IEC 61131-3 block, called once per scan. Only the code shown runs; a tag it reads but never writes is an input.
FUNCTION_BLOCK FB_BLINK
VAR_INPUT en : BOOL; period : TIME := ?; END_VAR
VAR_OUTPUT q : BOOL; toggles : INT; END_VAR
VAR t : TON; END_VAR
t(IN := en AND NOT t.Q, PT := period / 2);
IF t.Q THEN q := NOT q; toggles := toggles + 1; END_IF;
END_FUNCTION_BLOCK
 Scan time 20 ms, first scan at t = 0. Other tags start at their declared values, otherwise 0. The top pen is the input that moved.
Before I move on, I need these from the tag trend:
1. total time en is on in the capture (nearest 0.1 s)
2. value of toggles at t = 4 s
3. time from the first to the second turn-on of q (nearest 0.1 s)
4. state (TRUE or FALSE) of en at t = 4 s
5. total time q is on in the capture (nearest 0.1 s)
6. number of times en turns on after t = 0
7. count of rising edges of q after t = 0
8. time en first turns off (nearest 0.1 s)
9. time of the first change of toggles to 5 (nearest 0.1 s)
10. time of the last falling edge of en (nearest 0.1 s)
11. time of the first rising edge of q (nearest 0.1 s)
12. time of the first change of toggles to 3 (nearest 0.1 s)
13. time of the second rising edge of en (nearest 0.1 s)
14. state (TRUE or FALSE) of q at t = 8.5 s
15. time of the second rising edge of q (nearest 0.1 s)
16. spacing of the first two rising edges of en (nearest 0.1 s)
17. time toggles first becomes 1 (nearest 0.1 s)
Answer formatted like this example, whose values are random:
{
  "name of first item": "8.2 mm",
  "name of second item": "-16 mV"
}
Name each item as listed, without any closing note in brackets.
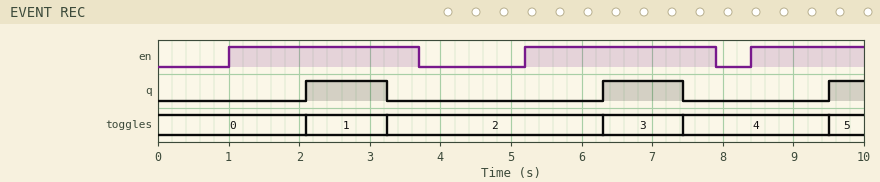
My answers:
{
  "total time en is on in the capture": "7.0 s",
  "value of toggles at t = 4 s": "2",
  "time from the first to the second turn-on of q": "4.2 s",
  "state (TRUE or FALSE) of en at t = 4 s": "FALSE",
  "total time q is on in the capture": "2.8 s",
  "number of times en turns on after t = 0": "3",
  "count of rising edges of q after t = 0": "3",
  "time en first turns off": "3.7 s",
  "time of the first change of toggles to 5": "9.5 s",
  "time of the last falling edge of en": "7.9 s",
  "time of the first rising edge of q": "2.1 s",
  "time of the first change of toggles to 3": "6.3 s",
  "time of the second rising edge of en": "5.2 s",
  "state (TRUE or FALSE) of q at t = 8.5 s": "FALSE",
  "time of the second rising edge of q": "6.3 s",
  "spacing of the first two rising edges of en": "4.2 s",
  "time toggles first becomes 1": "2.1 s"
}
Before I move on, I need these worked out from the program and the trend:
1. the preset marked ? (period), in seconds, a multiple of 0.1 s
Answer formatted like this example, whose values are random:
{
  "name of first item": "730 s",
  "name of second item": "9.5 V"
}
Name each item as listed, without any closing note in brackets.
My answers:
{
  "the preset marked ? (period), in seconds, a multiple of 0.1 s": "2.2 s"
}
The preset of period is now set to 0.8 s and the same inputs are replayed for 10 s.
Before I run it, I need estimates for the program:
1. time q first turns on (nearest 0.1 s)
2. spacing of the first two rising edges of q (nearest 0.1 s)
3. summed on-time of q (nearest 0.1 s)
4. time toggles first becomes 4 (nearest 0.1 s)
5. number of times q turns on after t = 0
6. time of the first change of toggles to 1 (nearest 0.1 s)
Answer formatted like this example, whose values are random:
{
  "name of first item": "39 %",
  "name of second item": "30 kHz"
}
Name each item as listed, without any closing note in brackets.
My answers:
{
  "time q first turns on": "1.4 s",
  "spacing of the first two rising edges of q": "0.9 s",
  "summed on-time of q": "3.4 s",
  "time toggles first becomes 4": "2.7 s",
  "number of times q turns on after t = 0": "8",
  "time of the first change of toggles to 1": "1.4 s"
}
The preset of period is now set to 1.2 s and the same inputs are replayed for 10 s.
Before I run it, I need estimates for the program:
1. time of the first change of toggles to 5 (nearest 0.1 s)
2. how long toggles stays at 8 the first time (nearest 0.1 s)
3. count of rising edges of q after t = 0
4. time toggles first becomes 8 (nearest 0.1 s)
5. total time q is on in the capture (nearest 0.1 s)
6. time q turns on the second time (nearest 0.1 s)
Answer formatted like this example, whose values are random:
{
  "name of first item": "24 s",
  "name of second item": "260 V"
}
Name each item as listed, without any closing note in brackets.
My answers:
{
  "time of the first change of toggles to 5": "5.8 s",
  "how long toggles stays at 8 the first time": "1.3 s",
  "count of rising edges of q after t = 0": "5",
  "time toggles first becomes 8": "7.7 s",
  "total time q is on in the capture": "3.2 s",
  "time q turns on the second time": "2.9 s"
}
